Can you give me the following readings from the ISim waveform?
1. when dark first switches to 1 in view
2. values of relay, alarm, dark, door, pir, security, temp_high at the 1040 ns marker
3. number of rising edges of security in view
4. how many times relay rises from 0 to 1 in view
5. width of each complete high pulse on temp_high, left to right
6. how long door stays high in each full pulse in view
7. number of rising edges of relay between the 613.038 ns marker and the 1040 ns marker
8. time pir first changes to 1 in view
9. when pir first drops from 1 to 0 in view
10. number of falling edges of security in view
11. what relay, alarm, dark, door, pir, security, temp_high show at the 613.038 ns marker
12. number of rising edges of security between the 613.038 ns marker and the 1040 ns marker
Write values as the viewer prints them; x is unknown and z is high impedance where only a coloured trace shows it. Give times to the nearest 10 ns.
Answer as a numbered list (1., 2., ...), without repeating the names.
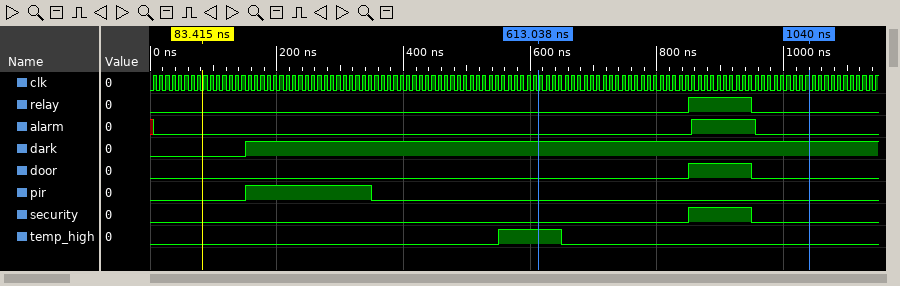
1. 150 ns
2. relay=0, alarm=0, dark=1, door=0, pir=0, security=0, temp_high=0
3. 1
4. 1
5. 100 ns
6. 100 ns
7. 1
8. 150 ns
9. 350 ns
10. 1
11. relay=0, alarm=0, dark=1, door=0, pir=0, security=0, temp_high=1
12. 1
